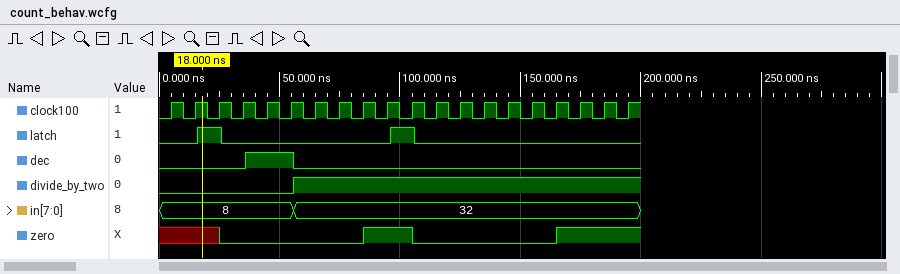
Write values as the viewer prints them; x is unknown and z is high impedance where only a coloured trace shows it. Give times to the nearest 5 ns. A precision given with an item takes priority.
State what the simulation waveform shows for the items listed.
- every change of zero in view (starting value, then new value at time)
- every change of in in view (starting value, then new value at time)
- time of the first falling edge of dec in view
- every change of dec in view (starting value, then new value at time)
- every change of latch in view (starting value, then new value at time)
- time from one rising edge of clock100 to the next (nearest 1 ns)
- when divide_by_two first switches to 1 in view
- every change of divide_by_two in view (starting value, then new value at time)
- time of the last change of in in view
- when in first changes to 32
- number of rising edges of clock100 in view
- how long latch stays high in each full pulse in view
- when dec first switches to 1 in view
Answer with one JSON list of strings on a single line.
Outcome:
["x, 0 at 25 ns, 1 at 85 ns, 0 at 105 ns, 1 at 165 ns", "8, 32 at 55 ns", "55 ns", "0, 1 at 35 ns, 0 at 55 ns", "0, 1 at 15 ns, 0 at 25 ns, 1 at 95 ns, 0 at 105 ns", "10 ns", "55 ns", "0, 1 at 55 ns", "55 ns", "55 ns", "20", "10 ns, 10 ns", "35 ns"]
